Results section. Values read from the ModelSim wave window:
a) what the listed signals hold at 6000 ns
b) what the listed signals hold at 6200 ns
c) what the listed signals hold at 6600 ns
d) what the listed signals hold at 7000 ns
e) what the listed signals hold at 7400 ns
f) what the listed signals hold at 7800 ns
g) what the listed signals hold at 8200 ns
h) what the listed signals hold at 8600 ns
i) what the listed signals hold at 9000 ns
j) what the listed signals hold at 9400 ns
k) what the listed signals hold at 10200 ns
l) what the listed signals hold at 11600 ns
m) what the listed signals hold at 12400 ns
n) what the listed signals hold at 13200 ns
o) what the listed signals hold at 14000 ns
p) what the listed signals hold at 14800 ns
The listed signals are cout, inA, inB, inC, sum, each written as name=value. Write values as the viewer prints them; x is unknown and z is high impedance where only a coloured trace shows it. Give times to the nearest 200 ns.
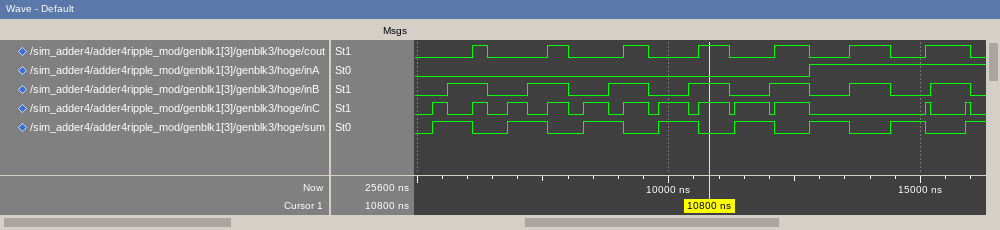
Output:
cout=0, inA=0, inB=1, inC=0, sum=1
cout=1, inA=0, inB=1, inC=1, sum=0
cout=0, inA=0, inB=0, inC=0, sum=0
cout=0, inA=0, inB=0, inC=1, sum=1
cout=0, inA=0, inB=1, inC=0, sum=1
cout=1, inA=0, inB=1, inC=1, sum=0
cout=0, inA=0, inB=0, inC=0, sum=0
cout=0, inA=0, inB=0, inC=1, sum=1
cout=0, inA=0, inB=1, inC=0, sum=1
cout=1, inA=0, inB=1, inC=1, sum=0
cout=0, inA=0, inB=0, inC=1, sum=1
cout=0, inA=0, inB=0, inC=1, sum=1
cout=1, inA=0, inB=1, inC=1, sum=0
cout=0, inA=1, inB=0, inC=0, sum=1
cout=1, inA=1, inB=1, inC=0, sum=0
cout=0, inA=1, inB=0, inC=0, sum=1
